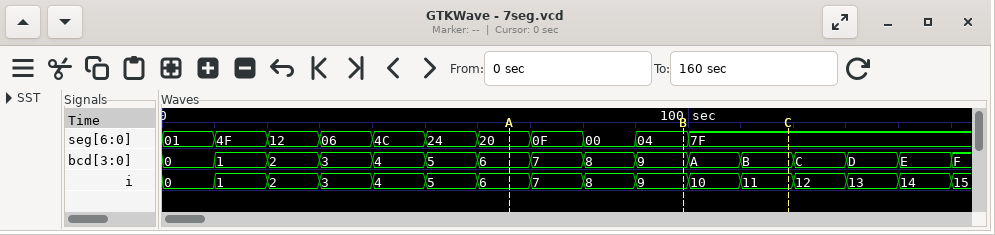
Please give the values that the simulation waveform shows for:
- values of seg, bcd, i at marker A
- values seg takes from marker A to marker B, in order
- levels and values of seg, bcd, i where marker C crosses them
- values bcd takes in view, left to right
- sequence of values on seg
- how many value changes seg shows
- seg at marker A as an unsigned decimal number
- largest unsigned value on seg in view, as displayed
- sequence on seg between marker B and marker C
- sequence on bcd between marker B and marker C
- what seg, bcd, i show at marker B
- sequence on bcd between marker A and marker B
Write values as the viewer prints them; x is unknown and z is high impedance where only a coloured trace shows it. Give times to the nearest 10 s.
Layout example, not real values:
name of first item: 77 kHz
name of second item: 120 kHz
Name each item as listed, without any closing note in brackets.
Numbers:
values of seg, bcd, i at marker A: seg=20, bcd=6, i=6
values seg takes from marker A to marker B, in order: 20, 0F, 00, 04
levels and values of seg, bcd, i where marker C crosses them: seg=7F, bcd=B, i=11
values bcd takes in view, left to right: 0, 1, 2, 3, 4, 5, 6, 7, 8, 9, A, B, C, D, E, F
sequence of values on seg: 01, 4F, 12, 06, 4C, 24, 20, 0F, 00, 04, 7F
how many value changes seg shows: 10
seg at marker A as an unsigned decimal number: 32
largest unsigned value on seg in view, as displayed: 7F
sequence on seg between marker B and marker C: 04, 7F
sequence on bcd between marker B and marker C: 9, A, B
what seg, bcd, i show at marker B: seg=04, bcd=9, i=9
sequence on bcd between marker A and marker B: 6, 7, 8, 9
